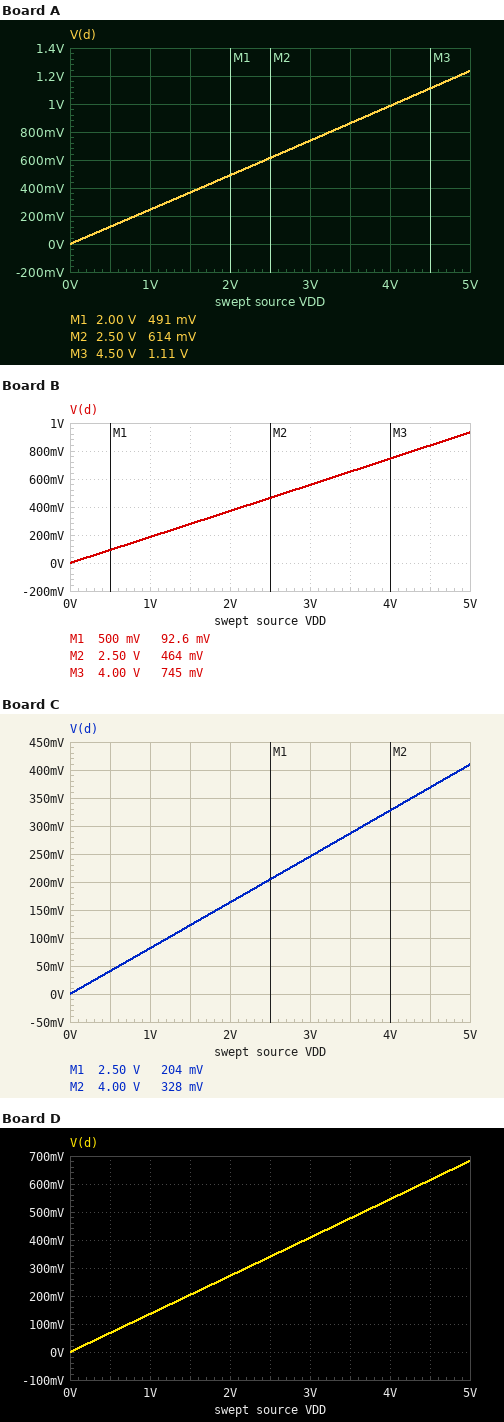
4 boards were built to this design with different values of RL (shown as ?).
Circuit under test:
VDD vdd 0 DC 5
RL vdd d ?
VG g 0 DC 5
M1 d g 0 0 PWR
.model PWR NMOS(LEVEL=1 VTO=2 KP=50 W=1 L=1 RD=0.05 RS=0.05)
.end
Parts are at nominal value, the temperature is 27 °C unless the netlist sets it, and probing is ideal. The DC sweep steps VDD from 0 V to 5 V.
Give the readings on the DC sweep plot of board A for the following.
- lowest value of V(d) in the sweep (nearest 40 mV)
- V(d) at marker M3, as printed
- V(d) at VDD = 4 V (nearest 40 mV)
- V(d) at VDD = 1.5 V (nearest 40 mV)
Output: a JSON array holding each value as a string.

["0 V", "1.11 V", "1.00 V", "360 mV"]
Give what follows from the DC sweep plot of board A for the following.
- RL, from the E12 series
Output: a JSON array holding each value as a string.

["0.33 Ω"]
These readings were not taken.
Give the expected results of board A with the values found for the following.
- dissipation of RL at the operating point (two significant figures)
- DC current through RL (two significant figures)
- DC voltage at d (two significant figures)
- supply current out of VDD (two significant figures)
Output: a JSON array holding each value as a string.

["43 W", "11 A", "1.2 V", "11 A"]
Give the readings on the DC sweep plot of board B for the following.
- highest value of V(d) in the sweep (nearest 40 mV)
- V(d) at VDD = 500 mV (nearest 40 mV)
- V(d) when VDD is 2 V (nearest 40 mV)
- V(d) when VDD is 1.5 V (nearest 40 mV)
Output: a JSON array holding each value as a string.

["920 mV", "80 mV", "360 mV", "280 mV"]
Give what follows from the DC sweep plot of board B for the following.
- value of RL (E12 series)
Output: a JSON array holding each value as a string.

["0.47 Ω"]
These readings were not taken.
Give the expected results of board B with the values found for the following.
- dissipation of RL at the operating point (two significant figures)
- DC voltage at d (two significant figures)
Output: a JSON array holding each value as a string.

["35 W", "930 mV"]
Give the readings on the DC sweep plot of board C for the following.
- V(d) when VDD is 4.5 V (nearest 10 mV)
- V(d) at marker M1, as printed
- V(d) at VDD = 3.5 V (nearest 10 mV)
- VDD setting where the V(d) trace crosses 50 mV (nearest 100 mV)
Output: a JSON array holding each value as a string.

["370 mV", "204 mV", "290 mV", "600 mV"]
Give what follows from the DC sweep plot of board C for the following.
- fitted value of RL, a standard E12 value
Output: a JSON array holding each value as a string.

["1.2 Ω"]
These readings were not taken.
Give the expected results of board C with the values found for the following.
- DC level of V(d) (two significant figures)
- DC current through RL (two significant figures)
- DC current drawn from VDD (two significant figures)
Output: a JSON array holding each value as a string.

["410 mV", "3.8 A", "3.8 A"]
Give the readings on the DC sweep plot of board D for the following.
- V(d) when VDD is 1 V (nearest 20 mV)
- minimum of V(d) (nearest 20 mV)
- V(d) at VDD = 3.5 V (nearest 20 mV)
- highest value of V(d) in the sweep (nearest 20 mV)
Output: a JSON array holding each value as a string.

["140 mV", "0 V", "480 mV", "680 mV"]
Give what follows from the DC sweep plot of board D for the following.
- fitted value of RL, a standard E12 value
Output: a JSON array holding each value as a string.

["0.68 Ω"]
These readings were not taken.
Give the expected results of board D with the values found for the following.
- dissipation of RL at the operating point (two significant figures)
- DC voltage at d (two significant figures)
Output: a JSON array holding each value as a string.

["27 W", "680 mV"]
